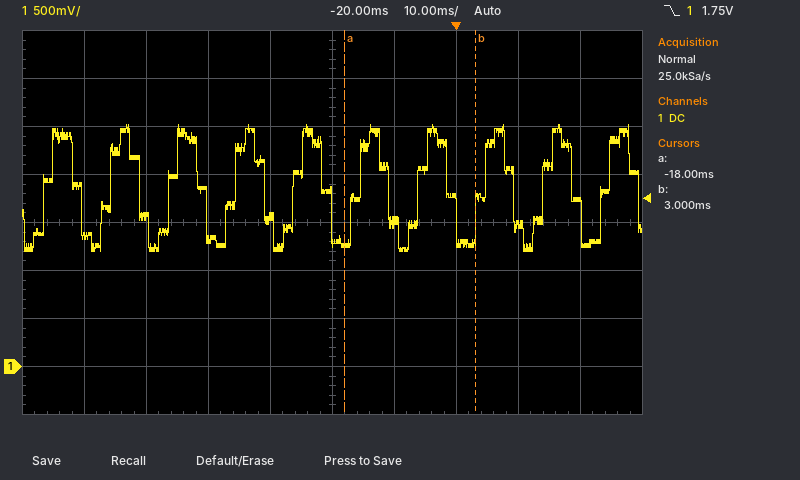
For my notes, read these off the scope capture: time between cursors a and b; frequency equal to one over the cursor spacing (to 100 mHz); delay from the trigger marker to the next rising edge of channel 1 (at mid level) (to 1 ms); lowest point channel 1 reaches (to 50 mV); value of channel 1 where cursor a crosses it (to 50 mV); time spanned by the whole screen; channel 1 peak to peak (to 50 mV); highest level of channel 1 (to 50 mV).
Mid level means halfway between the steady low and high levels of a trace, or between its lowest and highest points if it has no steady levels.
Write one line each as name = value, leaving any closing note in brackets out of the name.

time between cursors a and b = 21 ms
frequency equal to one over the cursor spacing = 47.6 Hz
delay from the trigger marker to the next rising edge of channel 1 (at mid level) = 5 ms
lowest point channel 1 reaches = 1.20 V
value of channel 1 where cursor a crosses it = 1.25 V
time spanned by the whole screen = 100 ms
channel 1 peak to peak = 1.30 V
highest level of channel 1 = 2.50 V
